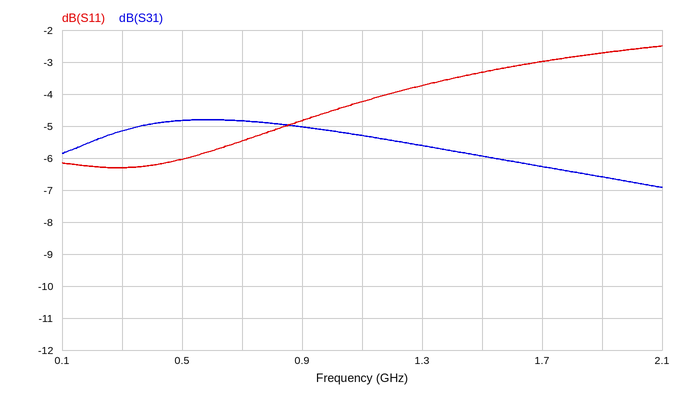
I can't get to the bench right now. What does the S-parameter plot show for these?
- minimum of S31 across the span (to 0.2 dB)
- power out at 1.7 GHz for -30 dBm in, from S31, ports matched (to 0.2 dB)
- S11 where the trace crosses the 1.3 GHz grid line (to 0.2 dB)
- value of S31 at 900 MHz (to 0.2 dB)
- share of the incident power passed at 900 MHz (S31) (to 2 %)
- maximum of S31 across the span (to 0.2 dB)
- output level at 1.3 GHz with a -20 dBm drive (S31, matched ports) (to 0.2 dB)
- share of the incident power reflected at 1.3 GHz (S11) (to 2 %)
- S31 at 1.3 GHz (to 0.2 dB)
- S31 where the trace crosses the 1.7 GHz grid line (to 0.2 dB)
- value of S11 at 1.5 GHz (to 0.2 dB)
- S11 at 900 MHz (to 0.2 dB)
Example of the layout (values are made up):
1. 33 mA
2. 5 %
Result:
1. -7.0 dB
2. -36.2 dBm
3. -3.8 dB
4. -5.0 dB
5. 32 %
6. -4.8 dB
7. -25.6 dBm
8. 42 %
9. -5.6 dB
10. -6.2 dB
11. -3.4 dB
12. -4.8 dB
